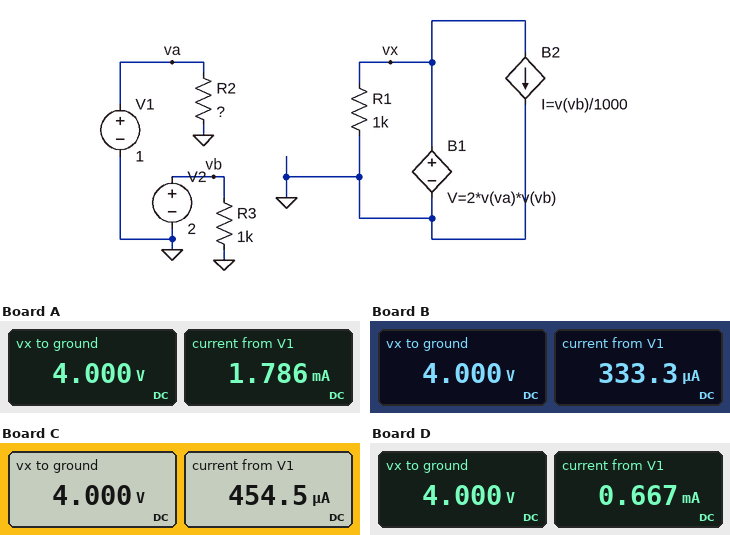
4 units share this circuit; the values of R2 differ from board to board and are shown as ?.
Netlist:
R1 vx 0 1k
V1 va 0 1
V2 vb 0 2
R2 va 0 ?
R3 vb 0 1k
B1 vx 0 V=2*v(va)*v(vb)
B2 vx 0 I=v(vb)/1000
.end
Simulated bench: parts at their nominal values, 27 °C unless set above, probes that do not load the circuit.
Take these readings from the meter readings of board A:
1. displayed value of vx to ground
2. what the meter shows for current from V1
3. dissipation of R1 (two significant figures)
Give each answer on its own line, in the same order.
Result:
4.000 V
1.786 mA
16 mW
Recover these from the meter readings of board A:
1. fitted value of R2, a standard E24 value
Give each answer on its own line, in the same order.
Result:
560 Ω
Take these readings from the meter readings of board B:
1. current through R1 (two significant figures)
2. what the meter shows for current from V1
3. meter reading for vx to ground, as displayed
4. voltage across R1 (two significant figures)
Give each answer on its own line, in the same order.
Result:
4.0 mA
333.3 µA
4.000 V
4.0 V
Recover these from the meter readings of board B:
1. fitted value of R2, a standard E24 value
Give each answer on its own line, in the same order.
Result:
3 kΩ
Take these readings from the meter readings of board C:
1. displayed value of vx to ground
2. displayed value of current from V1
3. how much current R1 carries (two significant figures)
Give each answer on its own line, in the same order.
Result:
4.000 V
454.5 µA
4.0 mA
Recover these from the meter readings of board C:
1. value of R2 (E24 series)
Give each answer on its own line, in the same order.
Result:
2.2 kΩ
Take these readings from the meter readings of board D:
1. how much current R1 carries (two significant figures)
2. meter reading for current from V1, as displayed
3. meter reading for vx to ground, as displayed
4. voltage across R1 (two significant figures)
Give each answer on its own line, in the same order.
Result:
4.0 mA
0.667 mA
4.000 V
4.0 V
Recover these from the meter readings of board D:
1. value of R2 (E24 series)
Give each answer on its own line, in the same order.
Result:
1.5 kΩ
